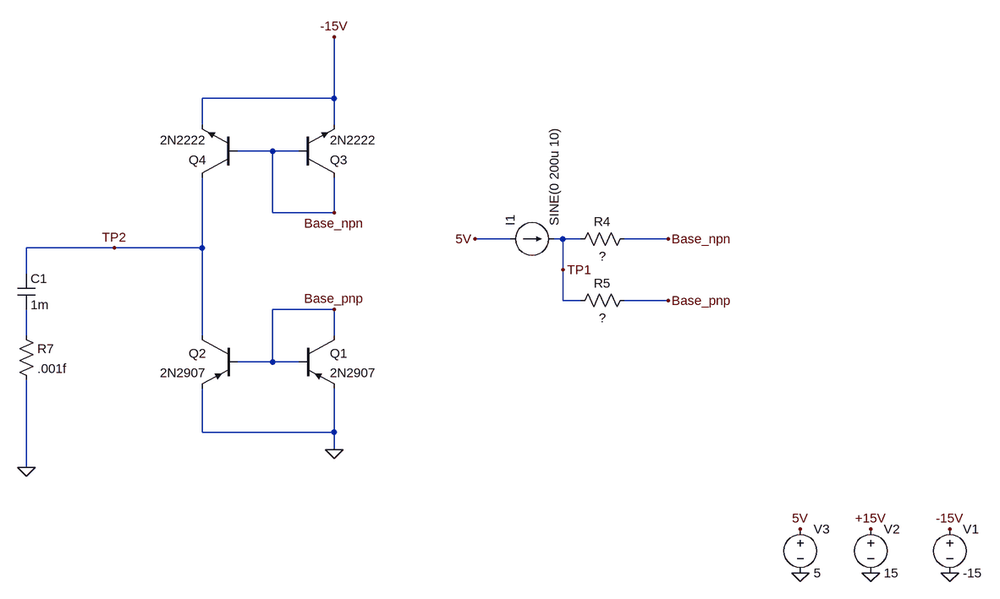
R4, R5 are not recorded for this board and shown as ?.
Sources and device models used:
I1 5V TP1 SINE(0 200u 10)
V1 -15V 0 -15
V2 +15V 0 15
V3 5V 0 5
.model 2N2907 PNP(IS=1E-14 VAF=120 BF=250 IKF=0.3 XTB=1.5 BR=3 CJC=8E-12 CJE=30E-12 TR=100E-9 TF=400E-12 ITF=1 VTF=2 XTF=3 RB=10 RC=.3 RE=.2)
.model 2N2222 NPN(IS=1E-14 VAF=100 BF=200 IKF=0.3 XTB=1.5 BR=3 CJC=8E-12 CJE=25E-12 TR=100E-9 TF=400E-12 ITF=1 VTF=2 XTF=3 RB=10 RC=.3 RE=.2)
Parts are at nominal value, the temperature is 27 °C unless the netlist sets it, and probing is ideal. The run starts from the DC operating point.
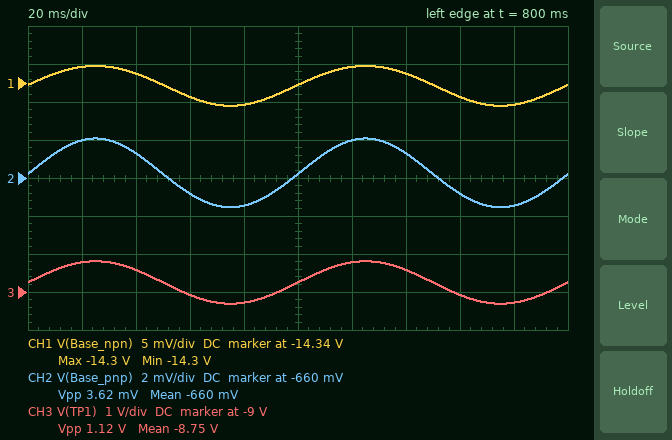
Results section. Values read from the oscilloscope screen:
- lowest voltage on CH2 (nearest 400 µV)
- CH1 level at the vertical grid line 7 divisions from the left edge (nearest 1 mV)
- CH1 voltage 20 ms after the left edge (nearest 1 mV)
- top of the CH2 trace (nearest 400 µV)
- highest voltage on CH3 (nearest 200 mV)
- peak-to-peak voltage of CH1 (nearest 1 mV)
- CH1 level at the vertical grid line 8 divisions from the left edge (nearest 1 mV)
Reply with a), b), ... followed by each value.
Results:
a) -661.6 mV
b) -14.339 V
c) -14.338 V
d) -658.0 mV
e) -8.2 V
f) 5 mV
g) -14.342 V
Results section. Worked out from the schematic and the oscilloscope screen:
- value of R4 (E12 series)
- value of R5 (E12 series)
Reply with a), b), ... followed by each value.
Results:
a) 4.7 kΩ
b) 6.8 kΩ
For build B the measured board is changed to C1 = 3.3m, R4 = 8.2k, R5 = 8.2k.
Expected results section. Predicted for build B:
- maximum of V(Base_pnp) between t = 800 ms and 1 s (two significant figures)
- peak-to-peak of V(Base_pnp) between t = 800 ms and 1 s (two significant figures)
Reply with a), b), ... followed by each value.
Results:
a) -650 mV
b) 6.3 mV
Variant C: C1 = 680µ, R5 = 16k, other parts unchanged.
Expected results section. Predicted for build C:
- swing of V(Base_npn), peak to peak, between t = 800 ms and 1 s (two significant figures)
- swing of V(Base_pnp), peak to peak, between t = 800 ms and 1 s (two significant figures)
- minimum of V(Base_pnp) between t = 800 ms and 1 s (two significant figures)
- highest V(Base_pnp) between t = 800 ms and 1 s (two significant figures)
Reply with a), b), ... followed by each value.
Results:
a) 12 mV
b) 3.6 mV
c) -650 mV
d) -640 mV
